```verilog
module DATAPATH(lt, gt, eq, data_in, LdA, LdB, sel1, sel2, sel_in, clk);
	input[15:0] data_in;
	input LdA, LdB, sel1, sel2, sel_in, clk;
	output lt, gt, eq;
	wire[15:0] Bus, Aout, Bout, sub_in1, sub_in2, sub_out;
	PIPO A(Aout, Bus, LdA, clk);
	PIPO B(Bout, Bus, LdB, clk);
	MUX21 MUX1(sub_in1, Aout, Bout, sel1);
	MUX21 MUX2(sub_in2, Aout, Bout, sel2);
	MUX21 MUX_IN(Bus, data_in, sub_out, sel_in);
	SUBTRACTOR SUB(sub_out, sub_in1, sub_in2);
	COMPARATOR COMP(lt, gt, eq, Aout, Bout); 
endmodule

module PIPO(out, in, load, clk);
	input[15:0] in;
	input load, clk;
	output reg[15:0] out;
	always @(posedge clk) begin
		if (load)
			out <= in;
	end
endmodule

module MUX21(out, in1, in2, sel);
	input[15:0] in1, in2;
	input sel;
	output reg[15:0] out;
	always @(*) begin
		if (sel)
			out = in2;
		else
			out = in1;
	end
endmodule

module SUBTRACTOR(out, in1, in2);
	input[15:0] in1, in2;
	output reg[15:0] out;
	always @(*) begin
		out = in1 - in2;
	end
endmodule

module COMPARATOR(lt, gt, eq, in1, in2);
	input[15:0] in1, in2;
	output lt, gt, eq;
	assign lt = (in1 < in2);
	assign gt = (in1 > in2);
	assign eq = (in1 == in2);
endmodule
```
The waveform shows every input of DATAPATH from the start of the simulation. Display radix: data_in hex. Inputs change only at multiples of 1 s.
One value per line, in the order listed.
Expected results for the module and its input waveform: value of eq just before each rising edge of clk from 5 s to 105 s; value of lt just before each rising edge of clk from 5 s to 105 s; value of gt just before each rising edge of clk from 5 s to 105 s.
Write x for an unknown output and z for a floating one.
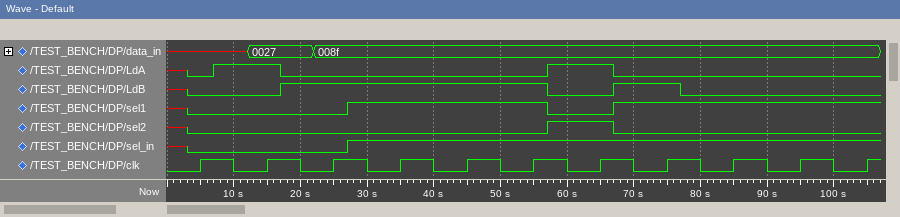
x x x 0 0 0 0 0 1 1 1
x x x 1 1 1 0 1 0 0 0
x x x 0 0 0 1 0 0 0 0
